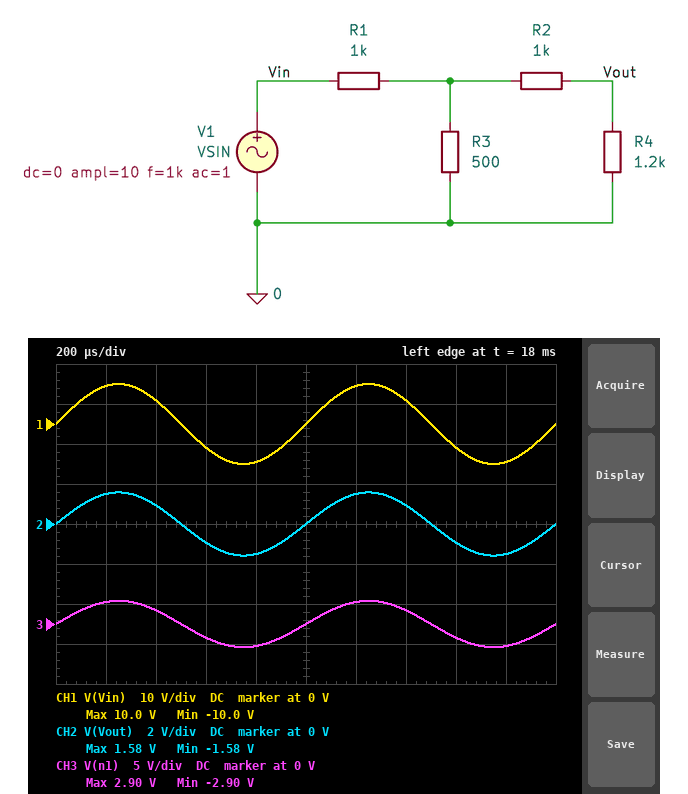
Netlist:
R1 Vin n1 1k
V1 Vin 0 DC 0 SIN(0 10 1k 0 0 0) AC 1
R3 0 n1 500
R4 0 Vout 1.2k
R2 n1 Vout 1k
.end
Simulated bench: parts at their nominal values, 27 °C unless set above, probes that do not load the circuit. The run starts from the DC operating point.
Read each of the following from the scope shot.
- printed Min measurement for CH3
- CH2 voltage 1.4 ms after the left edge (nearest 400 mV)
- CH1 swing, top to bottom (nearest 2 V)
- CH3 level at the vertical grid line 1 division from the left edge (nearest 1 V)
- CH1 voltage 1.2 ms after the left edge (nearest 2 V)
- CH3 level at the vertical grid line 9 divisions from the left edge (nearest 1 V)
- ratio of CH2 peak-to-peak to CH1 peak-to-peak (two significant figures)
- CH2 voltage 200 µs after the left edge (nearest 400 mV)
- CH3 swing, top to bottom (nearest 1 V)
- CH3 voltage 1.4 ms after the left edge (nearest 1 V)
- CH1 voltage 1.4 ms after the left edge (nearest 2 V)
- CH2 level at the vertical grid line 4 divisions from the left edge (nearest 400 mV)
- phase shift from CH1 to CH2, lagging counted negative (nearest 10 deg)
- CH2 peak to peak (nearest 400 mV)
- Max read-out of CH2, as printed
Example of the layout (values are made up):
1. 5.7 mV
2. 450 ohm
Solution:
1. -2.90 V
2. 800 mV
3. 20 V
4. 3 V
5. 10 V
6. -3 V
7. 0.16
8. 1.6 V
9. 6 V
10. 2 V
11. 6 V
12. -1.6 V
13. 0 deg
14. 3.2 V
15. 1.58 V
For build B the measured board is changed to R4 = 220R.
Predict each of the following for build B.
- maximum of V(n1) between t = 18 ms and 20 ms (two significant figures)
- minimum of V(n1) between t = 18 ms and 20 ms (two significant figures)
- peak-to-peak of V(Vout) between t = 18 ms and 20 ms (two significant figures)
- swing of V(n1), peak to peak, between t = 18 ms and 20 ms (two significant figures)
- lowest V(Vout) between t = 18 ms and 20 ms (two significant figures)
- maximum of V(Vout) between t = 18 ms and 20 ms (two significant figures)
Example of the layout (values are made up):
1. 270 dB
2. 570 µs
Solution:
1. 2.6 V
2. -2.6 V
3. 940 mV
4. 5.2 V
5. -470 mV
6. 470 mV
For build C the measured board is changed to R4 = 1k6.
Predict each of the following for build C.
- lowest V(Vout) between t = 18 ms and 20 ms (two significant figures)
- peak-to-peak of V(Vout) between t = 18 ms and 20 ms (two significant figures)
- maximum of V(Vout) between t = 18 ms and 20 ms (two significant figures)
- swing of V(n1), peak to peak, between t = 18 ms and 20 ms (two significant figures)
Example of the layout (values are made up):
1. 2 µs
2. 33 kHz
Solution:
1. -1.8 V
2. 3.6 V
3. 1.8 V
4. 5.9 V
